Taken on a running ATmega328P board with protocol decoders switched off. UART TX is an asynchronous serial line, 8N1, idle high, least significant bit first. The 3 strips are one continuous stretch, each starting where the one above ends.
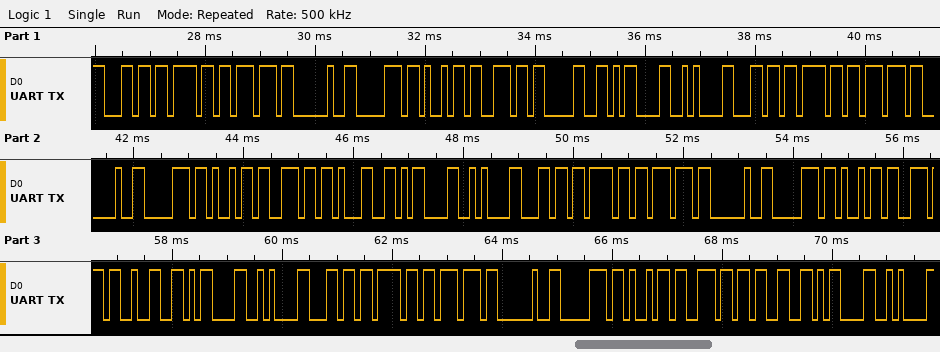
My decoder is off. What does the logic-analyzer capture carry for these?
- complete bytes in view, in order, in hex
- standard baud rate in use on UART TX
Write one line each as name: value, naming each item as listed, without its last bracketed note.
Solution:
complete bytes in view, in order, in hex: 6C 6F 77 20 70 69 6E 30 0D 0A 6C 6F 77 20 70 69 6E 31 0D 0A 6C 6F 77 20 70 69 6E 32 0D 0A 6C 6F 77 20 70 69 6E 33 0D 0A
standard baud rate in use on UART TX: 9600 baud
